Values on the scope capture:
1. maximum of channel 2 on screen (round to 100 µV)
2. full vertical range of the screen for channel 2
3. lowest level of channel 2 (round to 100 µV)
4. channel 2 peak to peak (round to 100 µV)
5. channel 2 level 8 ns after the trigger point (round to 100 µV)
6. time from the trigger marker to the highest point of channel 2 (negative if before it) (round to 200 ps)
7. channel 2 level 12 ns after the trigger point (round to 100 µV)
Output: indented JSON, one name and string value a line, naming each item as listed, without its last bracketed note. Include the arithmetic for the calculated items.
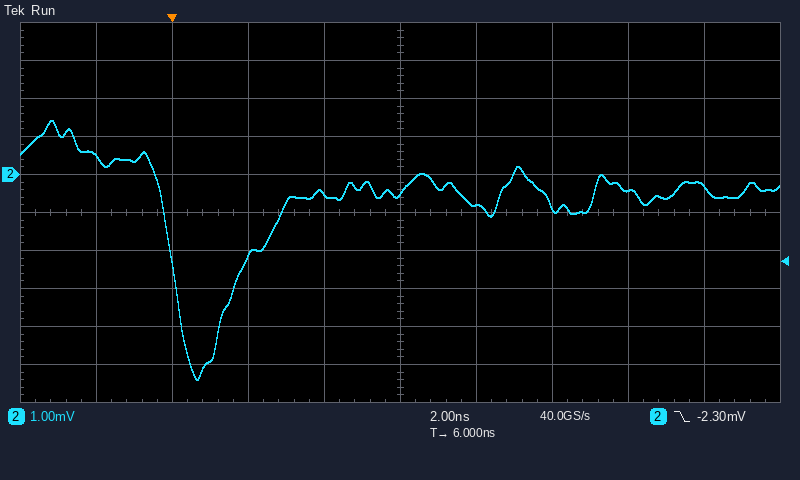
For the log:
{
  "maximum of channel 2 on screen": "1.4 mV",
  "full vertical range of the screen for channel 2": "10 mV",
  "lowest level of channel 2": "-5.4 mV",
  "channel 2 peak to peak": "1.4 mV − (-5.4 mV) = 6.8 mV",
  "channel 2 level 8 ns after the trigger point": "-800 µV",
  "time from the trigger marker to the highest point of channel 2 (negative if before it)": "-3.2 ns",
  "channel 2 level 12 ns after the trigger point": "-400 µV"
}
